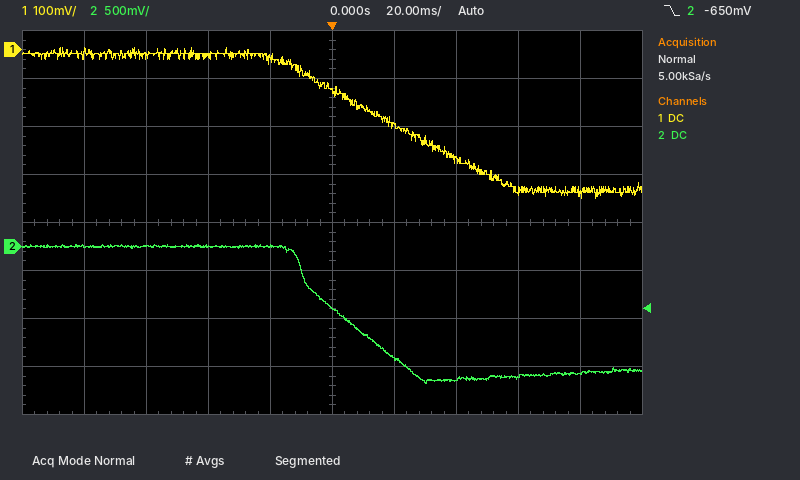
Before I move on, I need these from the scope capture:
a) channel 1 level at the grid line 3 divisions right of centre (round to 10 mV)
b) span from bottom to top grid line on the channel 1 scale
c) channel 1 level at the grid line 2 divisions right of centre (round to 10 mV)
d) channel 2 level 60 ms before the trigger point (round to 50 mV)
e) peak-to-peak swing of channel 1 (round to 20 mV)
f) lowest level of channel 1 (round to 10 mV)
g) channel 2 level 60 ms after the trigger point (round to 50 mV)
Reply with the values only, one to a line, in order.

-290 mV
800 mV
-230 mV
0 mV
320 mV
-310 mV
-1.35 V
